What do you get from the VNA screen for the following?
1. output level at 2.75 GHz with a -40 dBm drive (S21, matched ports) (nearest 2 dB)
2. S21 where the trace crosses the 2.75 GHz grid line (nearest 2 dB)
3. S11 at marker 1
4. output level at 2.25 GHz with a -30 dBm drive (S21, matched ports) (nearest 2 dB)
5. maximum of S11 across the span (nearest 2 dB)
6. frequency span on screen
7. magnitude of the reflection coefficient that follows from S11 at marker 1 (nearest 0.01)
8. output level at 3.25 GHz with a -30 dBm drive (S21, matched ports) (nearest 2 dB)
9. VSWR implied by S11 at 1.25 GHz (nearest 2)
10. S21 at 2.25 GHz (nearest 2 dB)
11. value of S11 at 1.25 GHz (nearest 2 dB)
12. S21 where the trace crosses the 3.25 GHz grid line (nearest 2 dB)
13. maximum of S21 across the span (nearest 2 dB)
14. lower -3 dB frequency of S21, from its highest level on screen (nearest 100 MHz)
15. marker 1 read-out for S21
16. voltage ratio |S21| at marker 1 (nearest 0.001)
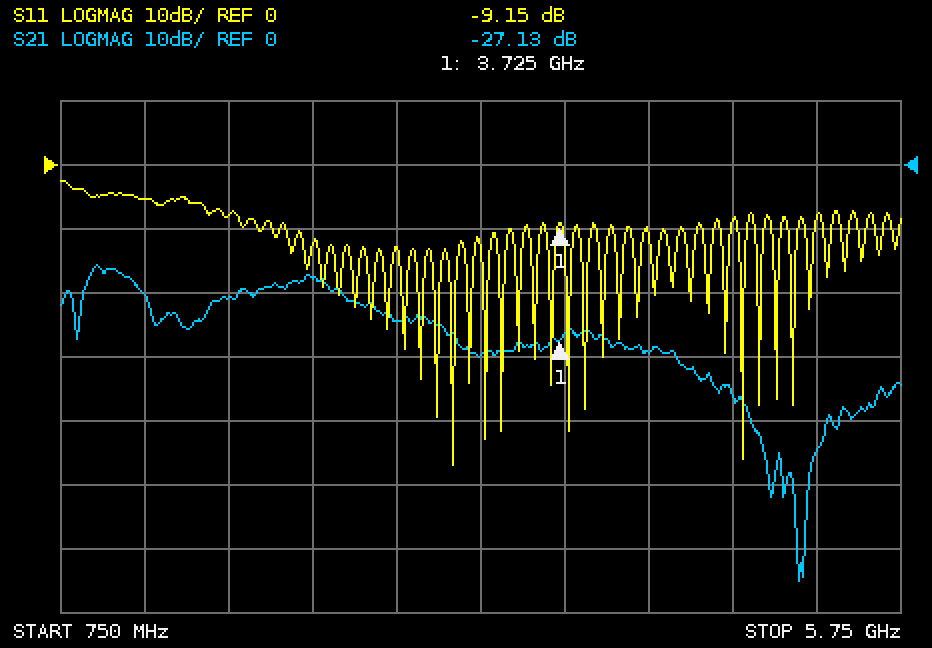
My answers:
-64 dBm
-24 dB
-9.15 dB
-48 dBm
-2 dB
5 GHz
0.35
-60 dBm
4
-18 dB
-6 dB
-30 dB
-16 dB
900 MHz
-27.13 dB
0.044
